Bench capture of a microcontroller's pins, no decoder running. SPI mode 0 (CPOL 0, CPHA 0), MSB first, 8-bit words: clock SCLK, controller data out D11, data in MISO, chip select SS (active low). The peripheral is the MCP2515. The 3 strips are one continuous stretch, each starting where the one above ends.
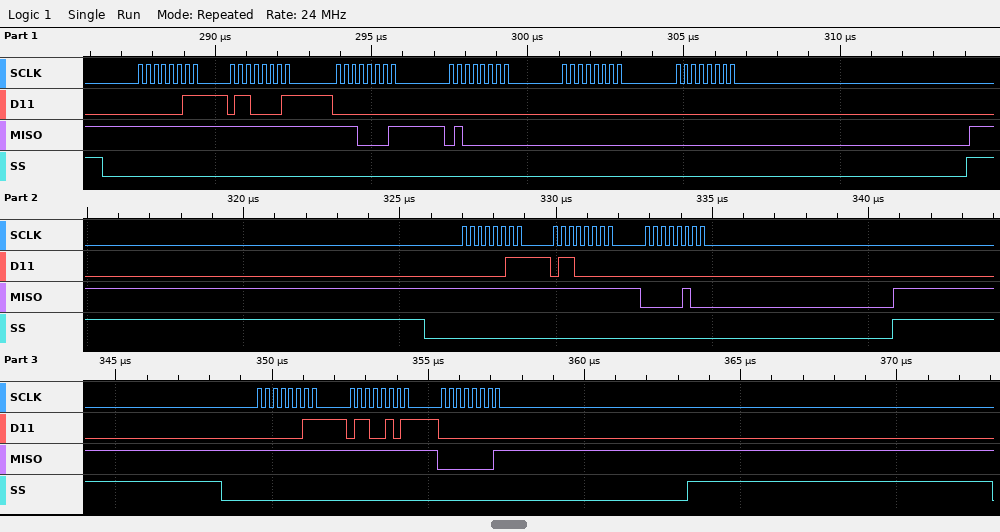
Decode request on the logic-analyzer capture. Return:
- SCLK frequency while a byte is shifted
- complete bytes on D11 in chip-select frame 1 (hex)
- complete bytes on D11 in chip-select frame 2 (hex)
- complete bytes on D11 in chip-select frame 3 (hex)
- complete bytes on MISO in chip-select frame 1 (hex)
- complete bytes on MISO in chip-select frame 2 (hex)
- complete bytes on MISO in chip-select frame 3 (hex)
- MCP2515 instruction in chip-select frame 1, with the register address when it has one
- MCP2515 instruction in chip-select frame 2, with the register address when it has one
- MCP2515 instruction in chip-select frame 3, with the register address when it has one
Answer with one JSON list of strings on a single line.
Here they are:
["4 MHz", "03 61 00 00 00 00", "03 60 00", "03 65 00", "FF FF E1 40 00 00", "FF FF 04", "FF FF 01", "READ 0x61", "READ 0x60", "READ 0x65"]
